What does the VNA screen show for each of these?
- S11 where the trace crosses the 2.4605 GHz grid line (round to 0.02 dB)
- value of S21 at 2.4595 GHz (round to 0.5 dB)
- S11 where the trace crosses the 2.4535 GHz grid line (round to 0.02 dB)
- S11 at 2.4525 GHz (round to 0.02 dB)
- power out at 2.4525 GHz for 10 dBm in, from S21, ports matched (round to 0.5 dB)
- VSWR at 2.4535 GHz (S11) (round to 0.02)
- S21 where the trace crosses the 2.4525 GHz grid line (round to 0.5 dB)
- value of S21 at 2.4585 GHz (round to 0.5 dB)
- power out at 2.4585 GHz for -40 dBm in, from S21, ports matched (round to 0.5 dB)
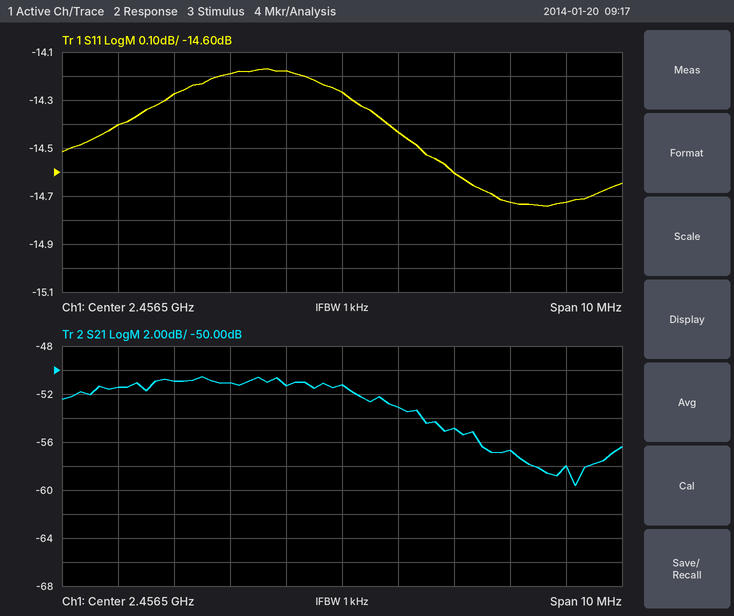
-14.72 dB
-56.5 dB
-14.28 dB
-14.40 dB
-41.5 dBm
1.48
-51.5 dB
-55.0 dB
-95.0 dBm
